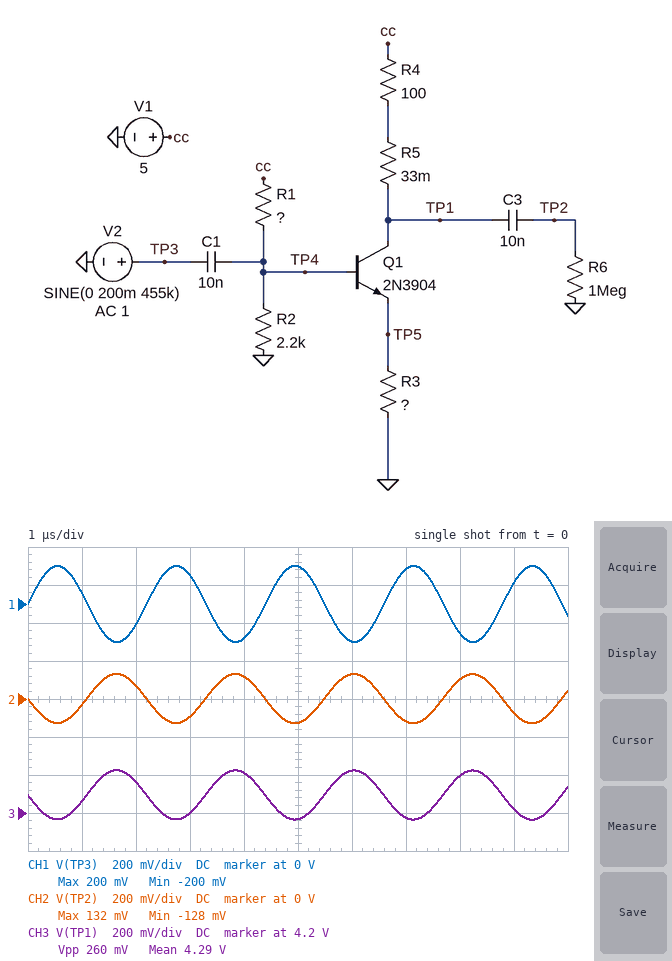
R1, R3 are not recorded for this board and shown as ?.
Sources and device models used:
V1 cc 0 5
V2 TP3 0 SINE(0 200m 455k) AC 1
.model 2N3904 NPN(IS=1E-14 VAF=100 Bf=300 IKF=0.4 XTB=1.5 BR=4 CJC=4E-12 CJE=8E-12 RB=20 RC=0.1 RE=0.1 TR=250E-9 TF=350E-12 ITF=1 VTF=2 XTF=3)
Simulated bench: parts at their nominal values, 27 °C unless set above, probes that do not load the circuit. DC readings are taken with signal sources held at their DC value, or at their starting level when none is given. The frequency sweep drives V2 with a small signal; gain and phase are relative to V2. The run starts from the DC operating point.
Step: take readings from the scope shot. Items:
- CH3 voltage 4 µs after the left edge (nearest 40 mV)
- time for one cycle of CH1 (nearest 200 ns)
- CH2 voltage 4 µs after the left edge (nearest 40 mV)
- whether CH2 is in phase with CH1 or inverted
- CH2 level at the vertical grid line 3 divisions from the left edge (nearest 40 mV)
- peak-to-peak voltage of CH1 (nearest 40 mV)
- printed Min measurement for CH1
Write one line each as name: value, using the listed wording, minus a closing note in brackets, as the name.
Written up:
CH3 voltage 4 µs after the left edge: 4.40 V
time for one cycle of CH1: 2.2 µs
CH2 voltage 4 µs after the left edge: 120 mV
whether CH2 is in phase with CH1 or inverted: inverted
CH2 level at the vertical grid line 3 divisions from the left edge: -80 mV
peak-to-peak voltage of CH1: 400 mV
printed Min measurement for CH1: -200 mV
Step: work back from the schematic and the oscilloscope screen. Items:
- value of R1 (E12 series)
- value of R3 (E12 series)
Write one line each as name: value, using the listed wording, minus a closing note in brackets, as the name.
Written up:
value of R1: 3.9 kΩ
value of R3: 150 Ω
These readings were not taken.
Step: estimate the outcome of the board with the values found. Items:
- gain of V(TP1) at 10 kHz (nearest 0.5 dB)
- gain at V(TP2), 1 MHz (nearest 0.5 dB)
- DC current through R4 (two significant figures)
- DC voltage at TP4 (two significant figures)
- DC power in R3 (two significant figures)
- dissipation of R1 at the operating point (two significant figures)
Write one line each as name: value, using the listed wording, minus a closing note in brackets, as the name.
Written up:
gain of V(TP1) at 10 kHz: -7.5 dB
gain at V(TP2), 1 MHz: -4.0 dB
DC current through R4: 7.1 mA
DC voltage at TP4: 1.8 V
DC power in R3: 7.5 mW
dissipation of R1 at the operating point: 2.7 mW
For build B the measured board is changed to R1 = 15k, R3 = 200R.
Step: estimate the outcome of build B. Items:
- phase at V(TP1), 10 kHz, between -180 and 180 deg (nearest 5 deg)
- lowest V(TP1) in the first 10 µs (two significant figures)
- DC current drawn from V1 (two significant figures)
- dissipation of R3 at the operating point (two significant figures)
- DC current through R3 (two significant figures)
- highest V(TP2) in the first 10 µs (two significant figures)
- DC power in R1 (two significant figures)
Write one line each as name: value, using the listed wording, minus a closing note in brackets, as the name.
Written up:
phase at V(TP1), 10 kHz, between -180 and 180 deg: -140 deg
lowest V(TP1) in the first 10 µs: 4.9 V
DC current drawn from V1: 450 µA
dissipation of R3 at the operating point: 5.1 µW
DC current through R3: 160 µA
highest V(TP2) in the first 10 µs: 16 mV
DC power in R1: 1.3 mW
